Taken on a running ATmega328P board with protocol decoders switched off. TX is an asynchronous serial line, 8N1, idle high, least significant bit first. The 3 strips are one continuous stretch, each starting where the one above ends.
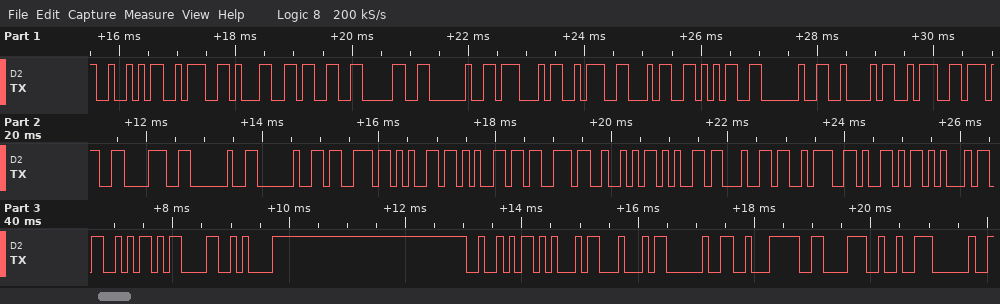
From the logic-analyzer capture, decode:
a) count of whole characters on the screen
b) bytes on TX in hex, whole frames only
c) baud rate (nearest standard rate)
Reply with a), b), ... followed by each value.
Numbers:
a) 38
b) 0x52 0x3A 0x31 0x33 0x30 0x20 0x47 0x3A 0x34 0x35 0x20 0x42 0x3A 0x37 0x38 0x20 0x20 0x73 0x65 0x65 0x73 0x52 0x65 0x64 0x3A 0x59 0x45 0x53 0x0D 0x0A 0x52 0x45 0x44 0x20 0xE2 0x86 0x92 0x20
c) 9600 baud
